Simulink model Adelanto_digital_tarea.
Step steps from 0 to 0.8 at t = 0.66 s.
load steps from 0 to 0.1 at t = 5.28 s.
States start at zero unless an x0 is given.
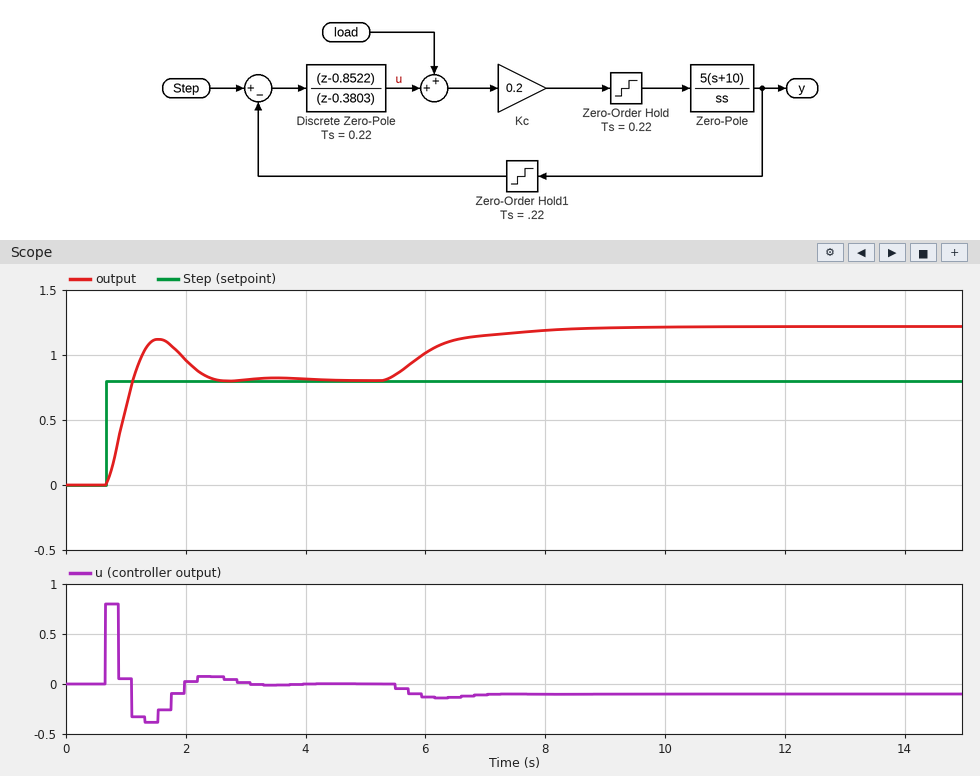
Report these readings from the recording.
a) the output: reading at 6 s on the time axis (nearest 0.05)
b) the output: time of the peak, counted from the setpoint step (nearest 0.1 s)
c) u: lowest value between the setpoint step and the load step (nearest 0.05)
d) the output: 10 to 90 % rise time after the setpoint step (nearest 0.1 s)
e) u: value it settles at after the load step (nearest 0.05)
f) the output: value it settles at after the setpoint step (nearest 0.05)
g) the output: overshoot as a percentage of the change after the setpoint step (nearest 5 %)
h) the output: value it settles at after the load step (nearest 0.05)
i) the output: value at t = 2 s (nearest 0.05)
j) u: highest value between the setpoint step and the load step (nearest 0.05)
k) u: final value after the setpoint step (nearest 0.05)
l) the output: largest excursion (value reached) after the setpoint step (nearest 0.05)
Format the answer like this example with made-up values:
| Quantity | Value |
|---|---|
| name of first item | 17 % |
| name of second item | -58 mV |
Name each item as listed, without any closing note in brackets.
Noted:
| Quantity | Value |
|---|---|
| the output: reading at 6 s on the time axis | 1.00 |
| the output: time of the peak, counted from the setpoint step | 0.9 s |
| u: lowest value between the setpoint step and the load step | -0.40 |
| the output: 10 to 90 % rise time after the setpoint step | 0.3 s |
| u: value it settles at after the load step | -0.10 |
| the output: value it settles at after the setpoint step | 0.80 |
| the output: overshoot as a percentage of the change after the setpoint step | 40 % |
| the output: value it settles at after the load step | 1.20 |
| the output: value at t = 2 s | 0.95 |
| u: highest value between the setpoint step and the load step | 0.80 |
| u: final value after the setpoint step | 0.00 |
| the output: largest excursion (value reached) after the setpoint step | 1.10 |
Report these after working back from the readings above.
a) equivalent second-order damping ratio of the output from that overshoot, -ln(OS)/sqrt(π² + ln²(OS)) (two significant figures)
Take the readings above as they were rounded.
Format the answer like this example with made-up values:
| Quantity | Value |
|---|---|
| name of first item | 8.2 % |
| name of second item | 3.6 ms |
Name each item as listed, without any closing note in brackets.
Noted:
| Quantity | Value |
|---|---|
| equivalent second-order damping ratio of the output from that overshoot, -ln(OS)/sqrt(π² + ln²(OS)) | 0.28 |
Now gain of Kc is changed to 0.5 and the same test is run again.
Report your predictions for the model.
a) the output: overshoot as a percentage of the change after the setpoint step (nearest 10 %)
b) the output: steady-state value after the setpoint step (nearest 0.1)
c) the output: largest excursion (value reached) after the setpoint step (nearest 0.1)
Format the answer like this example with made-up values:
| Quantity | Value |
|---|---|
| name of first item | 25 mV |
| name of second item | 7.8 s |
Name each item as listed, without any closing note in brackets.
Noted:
| Quantity | Value |
|---|---|
| the output: overshoot as a percentage of the change after the setpoint step | 60 % |
| the output: steady-state value after the setpoint step | 0.8 |
| the output: largest excursion (value reached) after the setpoint step | 1.3 |
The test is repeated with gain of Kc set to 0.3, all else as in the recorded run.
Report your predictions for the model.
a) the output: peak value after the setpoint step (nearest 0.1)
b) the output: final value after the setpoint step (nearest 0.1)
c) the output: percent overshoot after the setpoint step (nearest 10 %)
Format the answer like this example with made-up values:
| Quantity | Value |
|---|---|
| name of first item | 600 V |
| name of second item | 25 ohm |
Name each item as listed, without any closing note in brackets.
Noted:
| Quantity | Value |
|---|---|
| the output: peak value after the setpoint step | 1.2 |
| the output: final value after the setpoint step | 0.8 |
| the output: percent overshoot after the setpoint step | 50 % |
